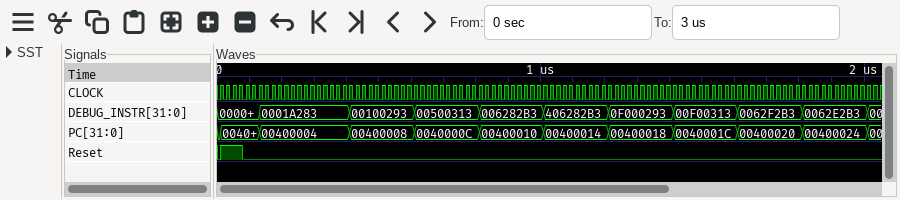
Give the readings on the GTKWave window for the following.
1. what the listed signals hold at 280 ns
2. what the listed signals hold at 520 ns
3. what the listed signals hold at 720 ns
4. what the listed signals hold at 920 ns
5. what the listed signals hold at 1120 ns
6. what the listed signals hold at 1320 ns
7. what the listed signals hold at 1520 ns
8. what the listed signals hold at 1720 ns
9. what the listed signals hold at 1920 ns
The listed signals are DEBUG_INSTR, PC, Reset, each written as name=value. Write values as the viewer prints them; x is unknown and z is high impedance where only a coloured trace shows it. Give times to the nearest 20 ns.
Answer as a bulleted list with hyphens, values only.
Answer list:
- DEBUG_INSTR=0001A283, PC=00400004, Reset=0
- DEBUG_INSTR=00100293, PC=00400008, Reset=0
- DEBUG_INSTR=00500313, PC=0040000C, Reset=0
- DEBUG_INSTR=006282B3, PC=00400010, Reset=0
- DEBUG_INSTR=406282B3, PC=00400014, Reset=0
- DEBUG_INSTR=0F000293, PC=00400018, Reset=0
- DEBUG_INSTR=00F00313, PC=0040001C, Reset=0
- DEBUG_INSTR=0062F2B3, PC=00400020, Reset=0
- DEBUG_INSTR=0062E2B3, PC=00400024, Reset=0
